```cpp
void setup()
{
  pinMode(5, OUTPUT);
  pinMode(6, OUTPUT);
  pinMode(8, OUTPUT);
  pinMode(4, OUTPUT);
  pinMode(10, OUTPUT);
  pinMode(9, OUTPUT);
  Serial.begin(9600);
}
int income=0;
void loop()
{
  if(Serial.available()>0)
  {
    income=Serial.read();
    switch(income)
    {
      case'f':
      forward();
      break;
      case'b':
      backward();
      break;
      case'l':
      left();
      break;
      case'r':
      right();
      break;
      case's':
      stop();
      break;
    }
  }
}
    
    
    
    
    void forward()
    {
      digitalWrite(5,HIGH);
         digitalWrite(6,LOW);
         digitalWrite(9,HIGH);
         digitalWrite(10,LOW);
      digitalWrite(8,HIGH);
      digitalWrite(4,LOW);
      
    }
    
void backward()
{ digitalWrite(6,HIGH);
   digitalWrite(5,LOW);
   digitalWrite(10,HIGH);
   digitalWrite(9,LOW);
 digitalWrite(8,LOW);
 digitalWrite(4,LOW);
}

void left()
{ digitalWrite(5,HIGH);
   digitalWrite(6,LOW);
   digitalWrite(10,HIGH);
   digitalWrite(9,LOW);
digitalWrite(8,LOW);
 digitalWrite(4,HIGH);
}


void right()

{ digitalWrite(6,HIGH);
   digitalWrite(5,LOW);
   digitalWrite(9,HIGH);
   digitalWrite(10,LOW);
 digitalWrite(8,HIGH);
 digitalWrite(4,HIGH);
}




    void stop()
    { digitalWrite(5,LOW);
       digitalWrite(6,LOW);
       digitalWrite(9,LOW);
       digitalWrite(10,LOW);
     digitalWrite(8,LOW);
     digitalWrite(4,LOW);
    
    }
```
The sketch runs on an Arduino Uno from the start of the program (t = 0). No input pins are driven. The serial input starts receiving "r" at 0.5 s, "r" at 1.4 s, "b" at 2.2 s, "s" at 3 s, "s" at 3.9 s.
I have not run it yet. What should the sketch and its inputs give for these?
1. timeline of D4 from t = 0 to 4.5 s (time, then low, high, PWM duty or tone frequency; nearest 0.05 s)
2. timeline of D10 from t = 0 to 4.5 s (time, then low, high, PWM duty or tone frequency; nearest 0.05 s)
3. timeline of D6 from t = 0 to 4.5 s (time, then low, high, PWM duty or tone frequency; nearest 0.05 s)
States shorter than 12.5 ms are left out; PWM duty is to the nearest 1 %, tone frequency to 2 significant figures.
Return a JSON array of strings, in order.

["0 s low; 0.5 s high; 2.2 s low", "0 s low; 2.2 s high; 3 s low", "0 s low; 0.5 s high; 3 s low"]
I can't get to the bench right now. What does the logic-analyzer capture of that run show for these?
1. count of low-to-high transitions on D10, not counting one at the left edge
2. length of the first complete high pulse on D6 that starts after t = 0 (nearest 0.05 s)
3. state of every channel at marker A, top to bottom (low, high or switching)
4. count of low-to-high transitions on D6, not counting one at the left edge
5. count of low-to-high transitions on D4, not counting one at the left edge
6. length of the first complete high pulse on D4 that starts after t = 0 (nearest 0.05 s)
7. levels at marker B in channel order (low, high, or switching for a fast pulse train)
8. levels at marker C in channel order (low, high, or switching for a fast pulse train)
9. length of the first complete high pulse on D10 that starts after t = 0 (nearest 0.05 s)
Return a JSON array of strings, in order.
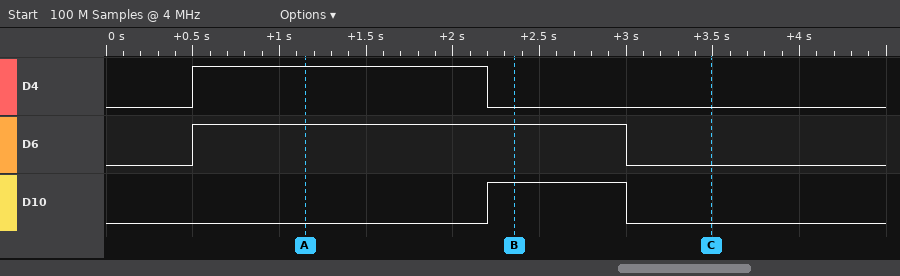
["1", "2.50 s", "D4 high, D6 high, D10 low", "1", "1", "1.70 s", "D4 low, D6 high, D10 high", "D4 low, D6 low, D10 low", "0.80 s"]
